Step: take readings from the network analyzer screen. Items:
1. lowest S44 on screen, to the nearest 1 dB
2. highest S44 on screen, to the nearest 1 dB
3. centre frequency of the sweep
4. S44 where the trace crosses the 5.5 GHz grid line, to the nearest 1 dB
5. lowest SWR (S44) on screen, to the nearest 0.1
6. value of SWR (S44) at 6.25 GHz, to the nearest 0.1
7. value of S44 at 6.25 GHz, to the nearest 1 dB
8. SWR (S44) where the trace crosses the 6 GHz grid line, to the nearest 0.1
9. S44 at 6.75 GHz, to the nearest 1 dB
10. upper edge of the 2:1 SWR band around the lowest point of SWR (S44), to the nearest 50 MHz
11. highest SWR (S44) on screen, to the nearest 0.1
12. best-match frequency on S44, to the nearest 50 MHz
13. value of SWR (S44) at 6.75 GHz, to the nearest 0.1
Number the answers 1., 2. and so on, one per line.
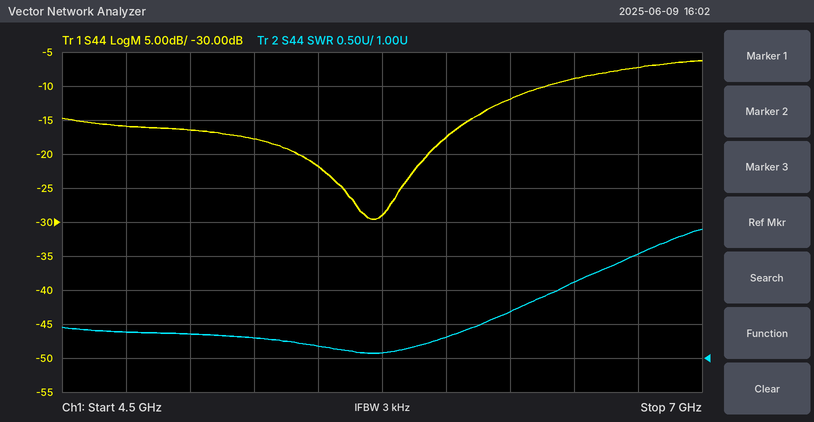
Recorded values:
1. -30 dB
2. -6 dB
3. 5.75 GHz
4. -22 dB
5. 1.1
6. 1.7
7. -12 dB
8. 1.3
9. -7 dB
10. 6.45 GHz
11. 2.9
12. 5.70 GHz
13. 2.5
